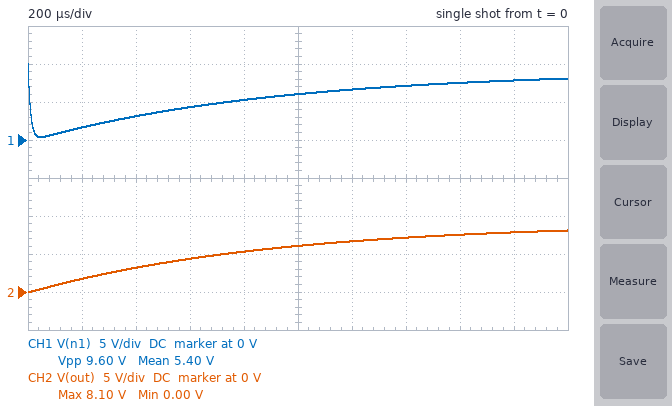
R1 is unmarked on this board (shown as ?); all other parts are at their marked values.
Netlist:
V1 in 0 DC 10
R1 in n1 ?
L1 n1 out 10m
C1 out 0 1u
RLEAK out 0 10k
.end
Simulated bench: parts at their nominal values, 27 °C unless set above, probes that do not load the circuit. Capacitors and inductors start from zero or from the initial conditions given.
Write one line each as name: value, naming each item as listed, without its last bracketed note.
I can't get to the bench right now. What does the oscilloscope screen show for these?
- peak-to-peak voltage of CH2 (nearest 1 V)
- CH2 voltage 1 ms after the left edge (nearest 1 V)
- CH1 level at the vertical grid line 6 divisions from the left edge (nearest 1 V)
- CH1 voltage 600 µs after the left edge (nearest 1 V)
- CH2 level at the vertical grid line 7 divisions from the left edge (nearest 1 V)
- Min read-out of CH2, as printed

peak-to-peak voltage of CH2: 8 V
CH2 voltage 1 ms after the left edge: 6 V
CH1 level at the vertical grid line 6 divisions from the left edge: 7 V
CH1 voltage 600 µs after the left edge: 4 V
CH2 level at the vertical grid line 7 divisions from the left edge: 7 V
Min read-out of CH2, as printed: 0.00 V
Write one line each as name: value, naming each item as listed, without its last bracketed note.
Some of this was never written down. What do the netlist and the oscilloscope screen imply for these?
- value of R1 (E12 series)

value of R1: 1 kΩ
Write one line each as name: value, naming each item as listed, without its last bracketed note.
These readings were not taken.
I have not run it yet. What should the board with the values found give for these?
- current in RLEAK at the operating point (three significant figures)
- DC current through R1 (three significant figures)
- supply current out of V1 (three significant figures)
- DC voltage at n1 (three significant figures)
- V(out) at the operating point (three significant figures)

current in RLEAK at the operating point: 909 µA
DC current through R1: 909 µA
supply current out of V1: 909 µA
DC voltage at n1: 9.09 V
V(out) at the operating point: 9.09 V
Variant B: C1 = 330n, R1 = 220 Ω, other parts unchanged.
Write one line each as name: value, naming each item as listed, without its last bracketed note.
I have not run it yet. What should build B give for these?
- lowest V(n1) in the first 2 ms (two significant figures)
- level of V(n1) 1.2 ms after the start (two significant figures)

lowest V(n1) in the first 2 ms: 3.9 V
level of V(n1) 1.2 ms after the start: 9.8 V
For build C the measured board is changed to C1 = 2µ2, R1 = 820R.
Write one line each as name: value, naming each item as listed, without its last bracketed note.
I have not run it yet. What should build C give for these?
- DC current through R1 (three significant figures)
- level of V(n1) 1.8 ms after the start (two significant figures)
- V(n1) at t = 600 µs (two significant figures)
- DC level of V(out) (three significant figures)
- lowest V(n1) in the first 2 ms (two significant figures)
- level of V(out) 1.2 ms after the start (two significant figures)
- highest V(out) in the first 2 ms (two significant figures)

DC current through R1: 924 µA
level of V(n1) 1.8 ms after the start: 6.1 V
V(n1) at t = 600 µs: 2.7 V
DC level of V(out): 9.24 V
lowest V(n1) in the first 2 ms: 270 mV
level of V(out) 1.2 ms after the start: 4.7 V
highest V(out) in the first 2 ms: 6.5 V
